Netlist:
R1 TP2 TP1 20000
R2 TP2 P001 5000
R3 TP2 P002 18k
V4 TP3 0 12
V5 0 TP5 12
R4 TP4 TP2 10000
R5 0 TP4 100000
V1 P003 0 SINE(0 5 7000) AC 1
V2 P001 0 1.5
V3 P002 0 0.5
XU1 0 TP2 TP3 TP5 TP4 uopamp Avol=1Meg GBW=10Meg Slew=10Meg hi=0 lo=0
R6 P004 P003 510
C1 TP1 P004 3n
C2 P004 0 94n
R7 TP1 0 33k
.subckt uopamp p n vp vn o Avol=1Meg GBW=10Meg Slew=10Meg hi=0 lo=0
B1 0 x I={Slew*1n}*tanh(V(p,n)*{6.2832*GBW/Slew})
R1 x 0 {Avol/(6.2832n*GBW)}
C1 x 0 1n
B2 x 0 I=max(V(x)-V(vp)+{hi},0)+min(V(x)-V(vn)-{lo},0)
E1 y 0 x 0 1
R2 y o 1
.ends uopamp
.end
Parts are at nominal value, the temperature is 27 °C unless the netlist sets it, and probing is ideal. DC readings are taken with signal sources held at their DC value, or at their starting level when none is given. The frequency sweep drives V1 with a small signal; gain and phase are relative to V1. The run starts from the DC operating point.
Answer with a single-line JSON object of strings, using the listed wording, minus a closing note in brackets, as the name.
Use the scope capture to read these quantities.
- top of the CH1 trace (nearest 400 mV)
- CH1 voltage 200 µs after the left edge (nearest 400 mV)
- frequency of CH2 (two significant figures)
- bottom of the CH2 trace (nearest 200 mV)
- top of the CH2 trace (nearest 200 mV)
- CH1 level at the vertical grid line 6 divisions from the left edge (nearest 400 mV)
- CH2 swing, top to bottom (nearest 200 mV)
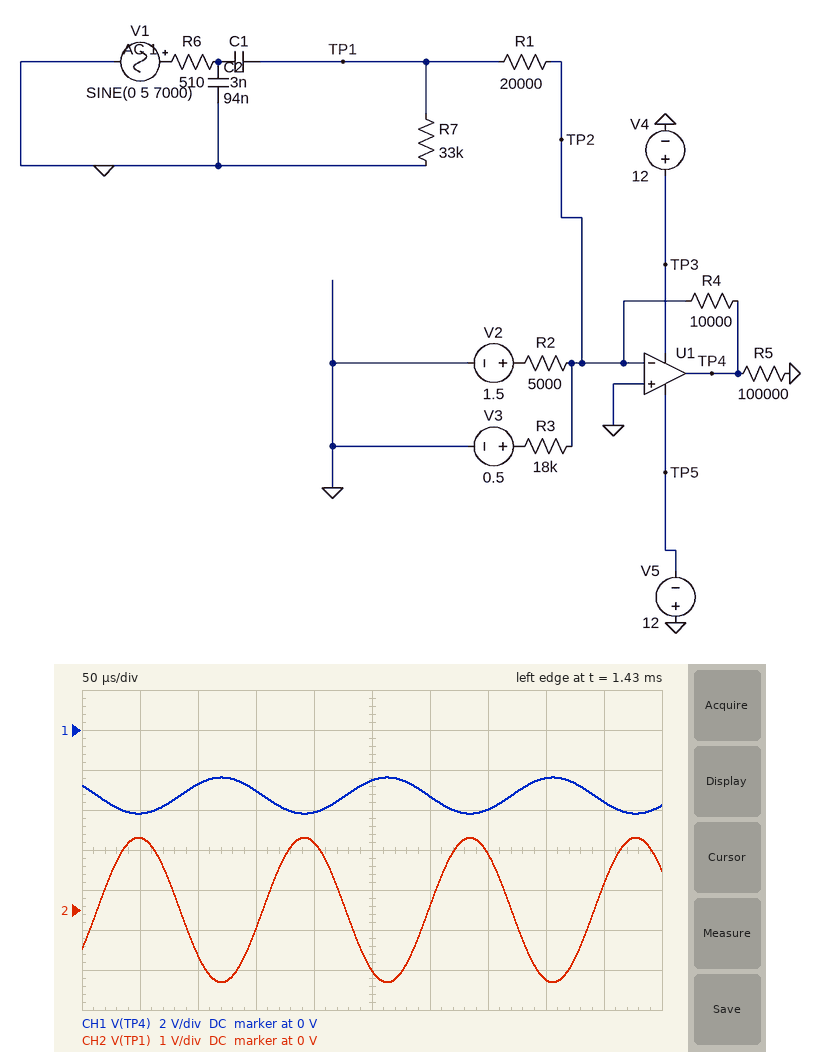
{"top of the CH1 trace": "-2.4 V", "CH1 voltage 200 µs after the left edge": "-4.0 V", "frequency of CH2": "7.0 kHz", "bottom of the CH2 trace": "-1.8 V", "top of the CH2 trace": "1.8 V", "CH1 level at the vertical grid line 6 divisions from the left edge": "-3.2 V", "CH2 swing, top to bottom": "3.6 V"}
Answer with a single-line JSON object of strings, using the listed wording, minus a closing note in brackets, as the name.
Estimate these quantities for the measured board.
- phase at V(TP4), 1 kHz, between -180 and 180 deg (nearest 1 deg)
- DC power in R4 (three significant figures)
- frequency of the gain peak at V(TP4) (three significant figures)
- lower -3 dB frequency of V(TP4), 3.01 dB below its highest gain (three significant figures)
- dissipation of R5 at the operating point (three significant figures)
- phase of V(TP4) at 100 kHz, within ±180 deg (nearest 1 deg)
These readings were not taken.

{"phase at V(TP4), 1 kHz, between -180 and 180 deg": "-120 deg", "DC power in R4": "1.07 mW", "frequency of the gain peak at V(TP4)": "3.76 kHz", "lower -3 dB frequency of V(TP4), 3.01 dB below its highest gain": "1.53 kHz", "dissipation of R5 at the operating point": "107 µW", "phase of V(TP4) at 100 kHz, within ±180 deg": "92 deg"}
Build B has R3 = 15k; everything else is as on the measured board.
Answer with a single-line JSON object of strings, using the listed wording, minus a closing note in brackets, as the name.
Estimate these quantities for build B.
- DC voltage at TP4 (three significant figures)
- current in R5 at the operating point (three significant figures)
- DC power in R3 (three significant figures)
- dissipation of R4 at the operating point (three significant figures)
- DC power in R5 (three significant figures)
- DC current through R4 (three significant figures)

{"DC voltage at TP4": "-3.33 V", "current in R5 at the operating point": "33.3 µA", "DC power in R3": "16.7 µW", "dissipation of R4 at the operating point": "1.11 mW", "DC power in R5": "111 µW", "DC current through R4": "333 µA"}
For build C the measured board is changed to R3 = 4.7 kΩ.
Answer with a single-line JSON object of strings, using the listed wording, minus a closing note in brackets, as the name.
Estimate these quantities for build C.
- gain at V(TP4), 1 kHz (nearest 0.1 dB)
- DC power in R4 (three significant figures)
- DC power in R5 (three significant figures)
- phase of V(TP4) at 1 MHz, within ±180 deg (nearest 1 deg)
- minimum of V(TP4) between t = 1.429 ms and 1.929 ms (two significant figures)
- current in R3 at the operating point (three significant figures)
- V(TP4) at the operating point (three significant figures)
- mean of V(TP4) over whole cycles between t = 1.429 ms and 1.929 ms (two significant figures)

{"gain at V(TP4), 1 kHz": "-19.3 dB", "DC power in R4": "1.65 mW", "DC power in R5": "165 µW", "phase of V(TP4) at 1 MHz, within ±180 deg": "61 deg", "minimum of V(TP4) between t = 1.429 ms and 1.929 ms": "-5.0 V", "current in R3 at the operating point": "106 µA", "V(TP4) at the operating point": "-4.06 V", "mean of V(TP4) over whole cycles between t = 1.429 ms and 1.929 ms": "-4.1 V"}
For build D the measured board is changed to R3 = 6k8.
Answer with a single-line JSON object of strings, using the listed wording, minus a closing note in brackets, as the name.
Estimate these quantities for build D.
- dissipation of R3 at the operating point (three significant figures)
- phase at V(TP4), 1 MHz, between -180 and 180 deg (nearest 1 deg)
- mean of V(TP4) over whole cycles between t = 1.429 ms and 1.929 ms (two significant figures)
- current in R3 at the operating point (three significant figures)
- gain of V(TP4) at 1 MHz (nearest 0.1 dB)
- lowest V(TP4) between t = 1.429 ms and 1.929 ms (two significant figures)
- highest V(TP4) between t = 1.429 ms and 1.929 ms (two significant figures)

{"dissipation of R3 at the operating point": "36.8 µW", "phase at V(TP4), 1 MHz, between -180 and 180 deg": "64 deg", "mean of V(TP4) over whole cycles between t = 1.429 ms and 1.929 ms": "-3.7 V", "current in R3 at the operating point": "73.5 µA", "gain of V(TP4) at 1 MHz": "-56.6 dB", "lowest V(TP4) between t = 1.429 ms and 1.929 ms": "-4.6 V", "highest V(TP4) between t = 1.429 ms and 1.929 ms": "-2.8 V"}
